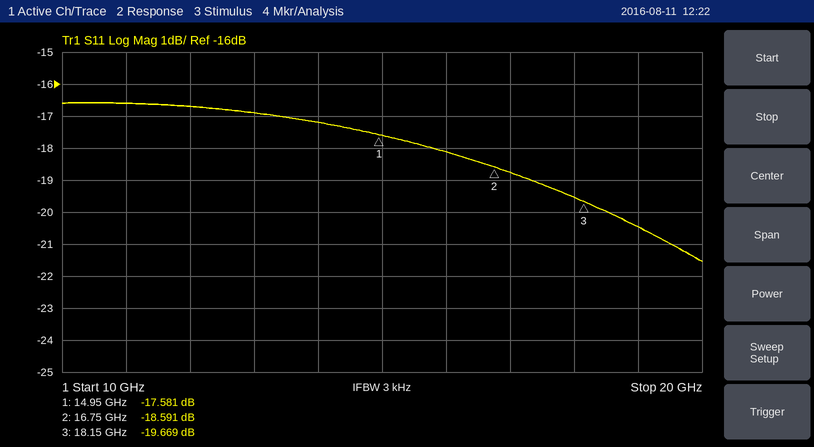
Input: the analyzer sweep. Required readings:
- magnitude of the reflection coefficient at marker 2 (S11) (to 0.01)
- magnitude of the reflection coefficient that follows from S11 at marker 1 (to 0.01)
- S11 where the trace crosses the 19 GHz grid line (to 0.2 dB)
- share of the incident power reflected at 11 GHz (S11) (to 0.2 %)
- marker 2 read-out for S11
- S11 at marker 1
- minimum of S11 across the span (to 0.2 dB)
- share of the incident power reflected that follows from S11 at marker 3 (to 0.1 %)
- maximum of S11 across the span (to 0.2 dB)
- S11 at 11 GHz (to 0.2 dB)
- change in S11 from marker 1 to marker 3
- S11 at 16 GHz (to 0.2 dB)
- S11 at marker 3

0.12
0.13
-20.4 dB
2.2 %
-18.591 dB
-17.581 dB
-21.6 dB
1.1 %
-16.6 dB
-16.6 dB
-2.088 dB
-18.2 dB
-19.669 dB
